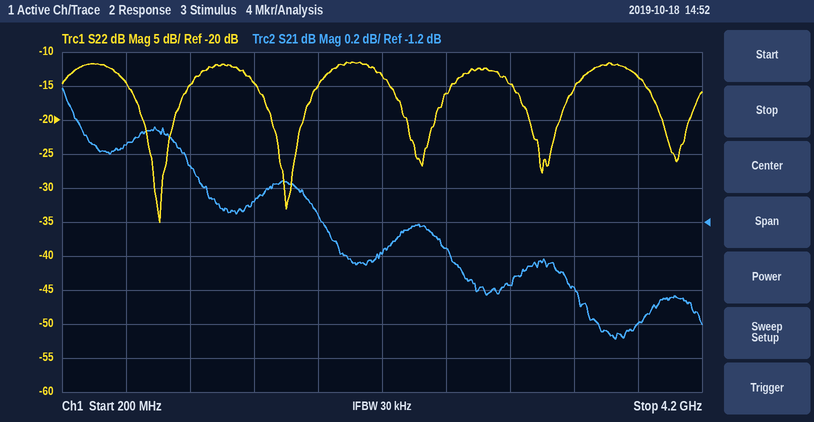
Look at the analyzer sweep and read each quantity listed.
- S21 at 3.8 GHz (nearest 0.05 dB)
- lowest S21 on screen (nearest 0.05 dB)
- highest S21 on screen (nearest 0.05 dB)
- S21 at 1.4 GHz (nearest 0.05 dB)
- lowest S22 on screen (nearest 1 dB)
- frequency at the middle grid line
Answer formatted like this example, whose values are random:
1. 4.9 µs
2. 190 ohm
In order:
1. -1.80 dB
2. -1.90 dB
3. -0.40 dB
4. -1.10 dB
5. -35 dB
6. 2.2 GHz
